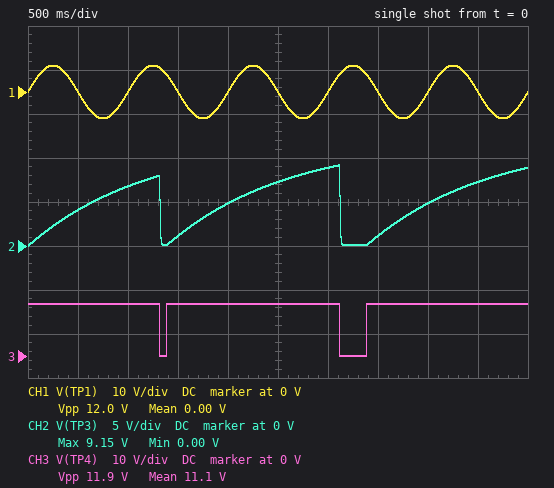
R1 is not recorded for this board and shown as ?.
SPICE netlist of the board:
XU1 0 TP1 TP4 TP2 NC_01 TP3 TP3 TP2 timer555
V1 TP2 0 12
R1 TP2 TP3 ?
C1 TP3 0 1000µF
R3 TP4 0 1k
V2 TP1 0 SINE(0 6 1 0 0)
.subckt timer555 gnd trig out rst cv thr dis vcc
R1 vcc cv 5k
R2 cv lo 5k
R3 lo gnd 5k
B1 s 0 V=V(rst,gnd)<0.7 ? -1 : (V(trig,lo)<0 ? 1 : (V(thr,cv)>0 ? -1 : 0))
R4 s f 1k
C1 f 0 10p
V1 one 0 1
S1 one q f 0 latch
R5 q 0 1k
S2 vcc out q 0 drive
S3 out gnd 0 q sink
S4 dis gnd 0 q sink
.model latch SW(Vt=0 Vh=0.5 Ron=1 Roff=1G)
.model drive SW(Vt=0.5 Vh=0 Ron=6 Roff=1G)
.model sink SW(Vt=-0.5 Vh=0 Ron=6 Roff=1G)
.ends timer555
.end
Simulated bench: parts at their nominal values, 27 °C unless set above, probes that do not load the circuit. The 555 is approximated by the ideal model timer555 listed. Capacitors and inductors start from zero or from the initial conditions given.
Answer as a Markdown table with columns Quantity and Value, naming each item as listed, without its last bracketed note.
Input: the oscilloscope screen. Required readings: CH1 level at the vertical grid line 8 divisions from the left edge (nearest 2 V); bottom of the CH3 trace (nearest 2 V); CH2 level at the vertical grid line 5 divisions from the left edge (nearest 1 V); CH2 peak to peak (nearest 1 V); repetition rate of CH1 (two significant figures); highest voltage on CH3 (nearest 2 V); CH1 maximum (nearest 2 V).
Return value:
| Quantity | Value |
|---|---|
| CH1 level at the vertical grid line 8 divisions from the left edge | 0 V |
| bottom of the CH3 trace | 0 V |
| CH2 level at the vertical grid line 5 divisions from the left edge | 7 V |
| CH2 peak to peak | 9 V |
| repetition rate of CH1 | 1.0 Hz |
| highest voltage on CH3 | 12 V |
| CH1 maximum | 6 V |
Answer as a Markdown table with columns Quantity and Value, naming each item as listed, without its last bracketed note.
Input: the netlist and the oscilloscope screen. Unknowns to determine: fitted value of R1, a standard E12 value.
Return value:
| Quantity | Value |
|---|---|
| fitted value of R1, a standard E12 value | 1.2 kΩ |
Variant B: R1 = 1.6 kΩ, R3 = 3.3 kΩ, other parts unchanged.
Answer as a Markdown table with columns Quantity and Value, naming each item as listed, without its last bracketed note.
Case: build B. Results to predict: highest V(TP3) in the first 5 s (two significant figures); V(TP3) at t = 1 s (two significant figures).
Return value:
| Quantity | Value |
|---|---|
| highest V(TP3) in the first 5 s | 8.8 V |
| V(TP3) at t = 1 s | 5.6 V |
